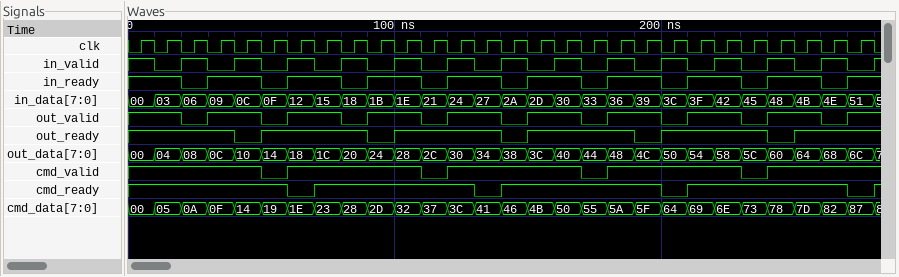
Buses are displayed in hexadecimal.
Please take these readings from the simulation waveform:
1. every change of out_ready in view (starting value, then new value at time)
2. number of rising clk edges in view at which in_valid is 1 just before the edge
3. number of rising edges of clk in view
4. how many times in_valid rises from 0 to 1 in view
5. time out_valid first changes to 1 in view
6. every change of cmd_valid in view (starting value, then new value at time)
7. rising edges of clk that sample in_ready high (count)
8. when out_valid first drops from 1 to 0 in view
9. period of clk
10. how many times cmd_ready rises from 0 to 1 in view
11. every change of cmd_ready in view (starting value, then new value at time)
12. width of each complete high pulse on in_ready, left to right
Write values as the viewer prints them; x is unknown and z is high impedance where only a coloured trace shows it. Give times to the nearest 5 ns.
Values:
1, 0 at 40 ns, 1 at 50 ns, 0 at 90 ns, 1 at 100 ns, 0 at 140 ns, 1 at 150 ns, 0 at 190 ns, 1 at 200 ns, 0 at 240 ns, 1 at 250 ns
14
28
14
30 ns
1, 0 at 50 ns, 1 at 60 ns, 0 at 110 ns, 1 at 120 ns, 0 at 170 ns, 1 at 180 ns, 0 at 230 ns, 1 at 240 ns
19
20 ns
10 ns
4
1, 0 at 60 ns, 1 at 70 ns, 0 at 130 ns, 1 at 140 ns, 0 at 200 ns, 1 at 210 ns, 0 at 270 ns, 1 at 280 ns
20 ns, 20 ns, 20 ns, 20 ns, 20 ns, 20 ns, 20 ns, 20 ns
